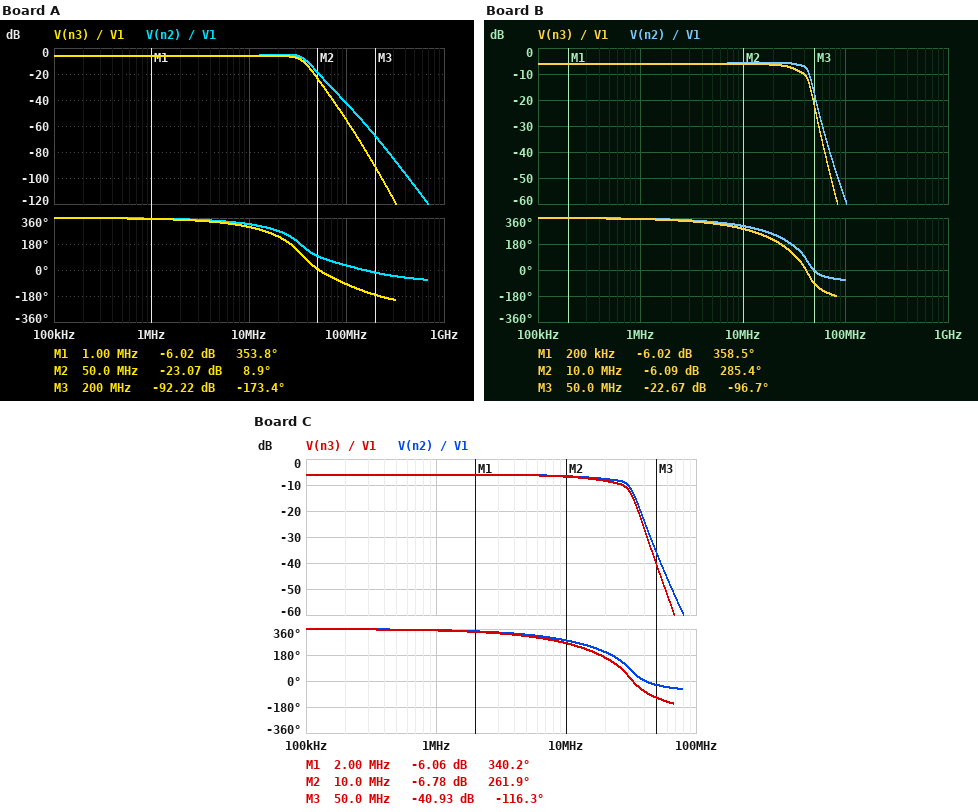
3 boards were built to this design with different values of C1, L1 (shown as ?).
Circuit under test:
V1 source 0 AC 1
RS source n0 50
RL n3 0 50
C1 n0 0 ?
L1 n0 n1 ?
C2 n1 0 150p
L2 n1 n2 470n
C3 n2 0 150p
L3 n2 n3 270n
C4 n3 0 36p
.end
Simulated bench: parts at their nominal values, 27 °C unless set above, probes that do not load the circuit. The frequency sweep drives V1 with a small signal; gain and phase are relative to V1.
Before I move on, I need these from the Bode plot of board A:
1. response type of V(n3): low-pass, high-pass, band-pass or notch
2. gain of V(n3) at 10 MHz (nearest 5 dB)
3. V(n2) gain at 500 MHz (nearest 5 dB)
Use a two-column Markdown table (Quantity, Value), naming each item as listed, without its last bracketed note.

| Quantity | Value |
|---|---|
| response type of V(n3): low-pass, high-pass, band-pass or notch | low-pass |
| gain of V(n3) at 10 MHz | -5 dB |
| V(n2) gain at 500 MHz | -105 dB |
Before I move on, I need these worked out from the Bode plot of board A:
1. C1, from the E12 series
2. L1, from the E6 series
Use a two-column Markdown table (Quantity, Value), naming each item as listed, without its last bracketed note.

| Quantity | Value |
|---|---|
| C1, from the E12 series | 12 pF |
| L1, from the E6 series | 100 nH |
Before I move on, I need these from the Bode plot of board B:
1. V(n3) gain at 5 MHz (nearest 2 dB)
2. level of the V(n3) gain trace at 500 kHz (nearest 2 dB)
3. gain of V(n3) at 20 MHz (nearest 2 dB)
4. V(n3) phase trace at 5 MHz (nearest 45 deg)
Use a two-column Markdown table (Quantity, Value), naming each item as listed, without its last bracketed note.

| Quantity | Value |
|---|---|
| V(n3) gain at 5 MHz | -6 dB |
| level of the V(n3) gain trace at 500 kHz | -6 dB |
| gain of V(n3) at 20 MHz | -6 dB |
| V(n3) phase trace at 5 MHz | 315 deg |
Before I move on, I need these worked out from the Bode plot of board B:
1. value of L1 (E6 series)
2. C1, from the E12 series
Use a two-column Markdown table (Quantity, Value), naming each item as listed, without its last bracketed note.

| Quantity | Value |
|---|---|
| value of L1 | 220 nH |
| C1, from the E12 series | 100 pF |
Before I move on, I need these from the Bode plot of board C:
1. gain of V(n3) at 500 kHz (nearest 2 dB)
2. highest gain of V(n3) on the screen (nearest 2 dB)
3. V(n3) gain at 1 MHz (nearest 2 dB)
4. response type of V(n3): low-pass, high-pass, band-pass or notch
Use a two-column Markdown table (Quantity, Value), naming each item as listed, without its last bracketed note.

| Quantity | Value |
|---|---|
| gain of V(n3) at 500 kHz | -6 dB |
| highest gain of V(n3) on the screen | -6 dB |
| V(n3) gain at 1 MHz | -6 dB |
| response type of V(n3): low-pass, high-pass, band-pass or notch | low-pass |
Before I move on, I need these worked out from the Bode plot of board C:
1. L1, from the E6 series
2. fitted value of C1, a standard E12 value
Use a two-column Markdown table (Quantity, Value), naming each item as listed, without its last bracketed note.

| Quantity | Value |
|---|---|
| L1, from the E6 series | 1 µH |
| fitted value of C1, a standard E12 value | 68 pF |
